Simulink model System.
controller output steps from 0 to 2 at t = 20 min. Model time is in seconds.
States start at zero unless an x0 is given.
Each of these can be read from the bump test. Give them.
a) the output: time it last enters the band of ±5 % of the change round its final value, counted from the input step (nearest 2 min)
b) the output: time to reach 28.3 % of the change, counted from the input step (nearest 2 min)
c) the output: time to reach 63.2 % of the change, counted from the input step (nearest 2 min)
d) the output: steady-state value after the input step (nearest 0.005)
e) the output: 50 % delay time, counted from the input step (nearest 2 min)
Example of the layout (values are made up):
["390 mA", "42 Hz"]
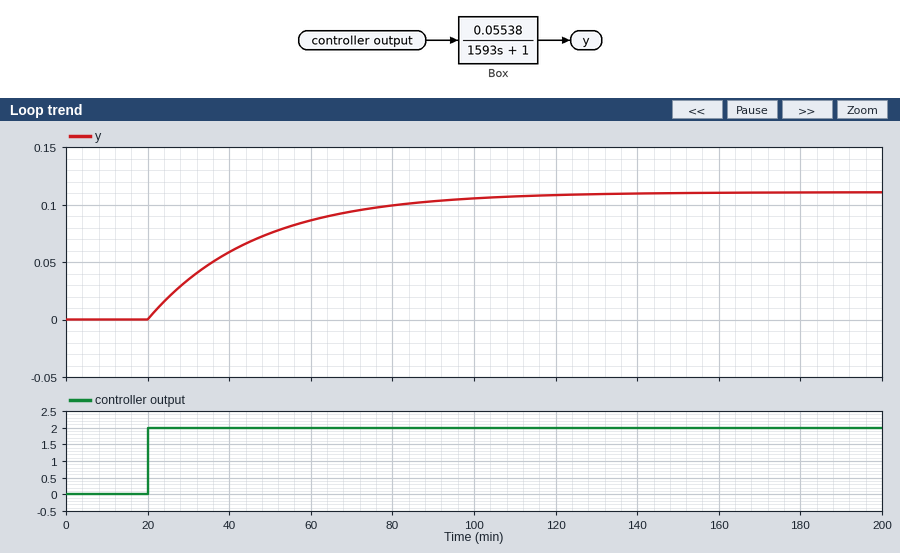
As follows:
["80 min", "8 min", "26 min", "0.110", "18 min"]
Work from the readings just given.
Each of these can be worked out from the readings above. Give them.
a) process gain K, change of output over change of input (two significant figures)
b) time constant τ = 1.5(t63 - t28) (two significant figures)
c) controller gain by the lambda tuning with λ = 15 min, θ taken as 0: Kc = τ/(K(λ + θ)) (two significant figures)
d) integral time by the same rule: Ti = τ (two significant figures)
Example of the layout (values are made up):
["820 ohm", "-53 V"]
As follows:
["0.055", "27 min", "33", "27 min"]
